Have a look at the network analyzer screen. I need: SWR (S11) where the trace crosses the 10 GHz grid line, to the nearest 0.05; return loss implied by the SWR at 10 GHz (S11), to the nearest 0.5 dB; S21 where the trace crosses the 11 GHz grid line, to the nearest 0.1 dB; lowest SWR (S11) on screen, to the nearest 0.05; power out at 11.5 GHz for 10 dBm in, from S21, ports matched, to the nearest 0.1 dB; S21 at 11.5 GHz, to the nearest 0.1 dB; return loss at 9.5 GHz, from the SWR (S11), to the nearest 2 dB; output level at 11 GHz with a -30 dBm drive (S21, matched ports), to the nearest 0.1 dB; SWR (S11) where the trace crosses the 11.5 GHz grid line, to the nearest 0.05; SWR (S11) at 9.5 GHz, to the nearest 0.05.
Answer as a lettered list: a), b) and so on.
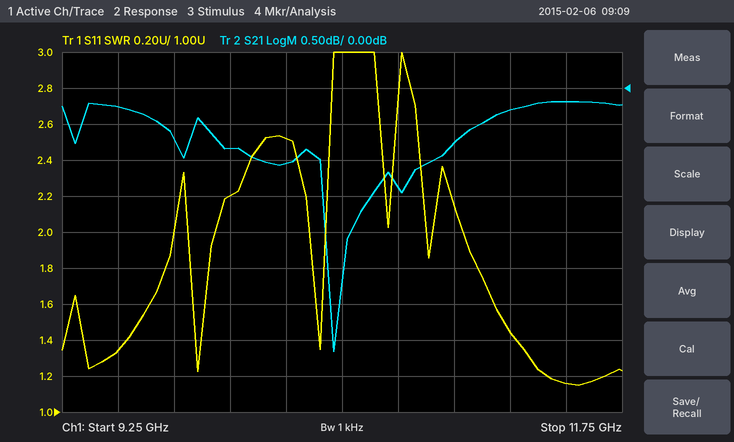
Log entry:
a) 2.20
b) 8.5 dB
c) -0.8 dB
d) 1.15
e) 9.8 dBm
f) -0.2 dB
g) 16 dB
h) -30.8 dBm
i) 1.15
j) 1.35
